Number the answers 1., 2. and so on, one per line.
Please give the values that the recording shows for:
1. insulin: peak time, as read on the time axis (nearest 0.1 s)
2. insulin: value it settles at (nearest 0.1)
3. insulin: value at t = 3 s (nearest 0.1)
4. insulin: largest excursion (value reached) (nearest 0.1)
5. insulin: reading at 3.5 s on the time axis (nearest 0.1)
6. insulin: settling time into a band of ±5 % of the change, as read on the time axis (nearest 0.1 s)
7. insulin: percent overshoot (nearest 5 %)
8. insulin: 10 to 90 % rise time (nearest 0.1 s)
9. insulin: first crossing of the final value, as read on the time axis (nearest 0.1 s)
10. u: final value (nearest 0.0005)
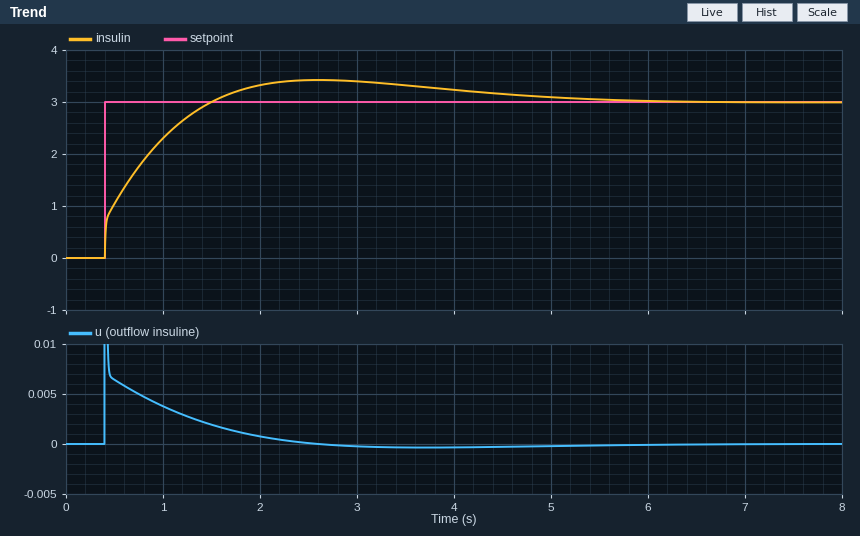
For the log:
1. 2.6 s
2. 3.0
3. 3.4
4. 3.4
5. 3.3
6. 4.5 s
7. 15 %
8. 0.8 s
9. 1.5 s
10. 0.0000
